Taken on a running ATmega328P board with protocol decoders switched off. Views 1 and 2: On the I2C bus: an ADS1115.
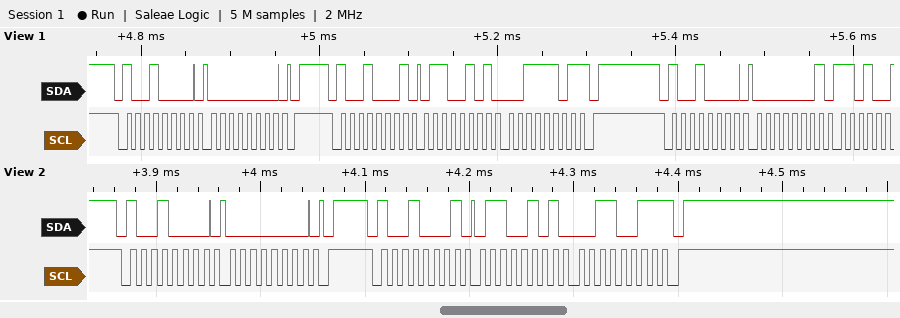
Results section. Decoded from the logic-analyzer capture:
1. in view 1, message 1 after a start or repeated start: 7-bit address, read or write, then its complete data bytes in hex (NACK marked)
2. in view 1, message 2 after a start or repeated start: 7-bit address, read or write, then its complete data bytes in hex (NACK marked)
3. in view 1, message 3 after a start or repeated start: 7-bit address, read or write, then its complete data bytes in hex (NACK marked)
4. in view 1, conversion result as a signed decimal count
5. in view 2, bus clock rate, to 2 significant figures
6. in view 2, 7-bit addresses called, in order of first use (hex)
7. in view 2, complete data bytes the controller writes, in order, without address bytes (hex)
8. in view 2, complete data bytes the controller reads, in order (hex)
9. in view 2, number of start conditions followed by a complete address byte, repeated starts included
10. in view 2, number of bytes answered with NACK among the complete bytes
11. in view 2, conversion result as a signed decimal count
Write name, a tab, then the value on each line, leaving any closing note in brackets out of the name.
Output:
in view 1, message 1 after a start or repeated start: 7-bit address, read or write, then its complete data bytes in hex	0x48 write: 00
in view 1, message 2 after a start or repeated start: 7-bit address, read or write, then its complete data bytes in hex	0x48 read: 65 3D NACK
in view 1, message 3 after a start or repeated start: 7-bit address, read or write, then its complete data bytes in hex	0x48 write: 01
in view 1, conversion result as a signed decimal count	25917
in view 2, bus clock rate, to 2 significant figures	100 kHz
in view 2, 7-bit addresses called, in order of first use	0x48
in view 2, complete data bytes the controller writes, in order, without address bytes	00
in view 2, complete data bytes the controller reads, in order	65 33
in view 2, number of start conditions followed by a complete address byte, repeated starts included	2
in view 2, number of bytes answered with NACK among the complete bytes	1
in view 2, conversion result as a signed decimal count	25907
